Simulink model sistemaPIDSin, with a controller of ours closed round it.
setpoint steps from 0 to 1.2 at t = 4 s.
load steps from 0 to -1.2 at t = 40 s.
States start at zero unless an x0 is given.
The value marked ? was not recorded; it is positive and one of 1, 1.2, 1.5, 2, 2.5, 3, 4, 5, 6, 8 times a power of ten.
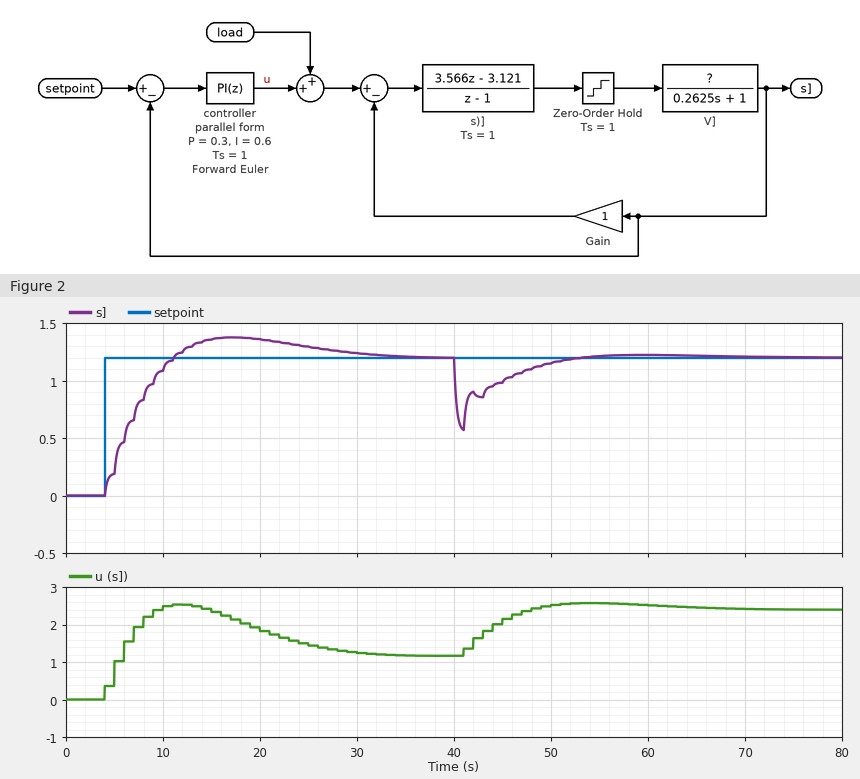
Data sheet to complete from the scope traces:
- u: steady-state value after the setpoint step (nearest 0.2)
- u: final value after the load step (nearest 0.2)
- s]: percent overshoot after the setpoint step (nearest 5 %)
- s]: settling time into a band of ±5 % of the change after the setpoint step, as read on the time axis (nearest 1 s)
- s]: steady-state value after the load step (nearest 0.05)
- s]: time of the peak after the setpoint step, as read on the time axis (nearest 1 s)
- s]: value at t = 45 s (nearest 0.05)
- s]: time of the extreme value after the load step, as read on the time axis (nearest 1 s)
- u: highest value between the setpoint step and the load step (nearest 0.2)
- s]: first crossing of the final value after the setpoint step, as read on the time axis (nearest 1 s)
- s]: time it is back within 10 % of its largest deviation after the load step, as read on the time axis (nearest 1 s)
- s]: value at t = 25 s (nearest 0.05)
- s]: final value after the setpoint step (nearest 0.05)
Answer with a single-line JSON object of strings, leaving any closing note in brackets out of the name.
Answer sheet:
{"u: steady-state value after the setpoint step": "1.2", "u: final value after the load step": "2.4", "s]: percent overshoot after the setpoint step": "15 %", "s]: settling time into a band of ±5 % of the change after the setpoint step, as read on the time axis": "28 s", "s]: steady-state value after the load step": "1.20", "s]: time of the peak after the setpoint step, as read on the time axis": "17 s", "s]: value at t = 45 s": "1.00", "s]: time of the extreme value after the load step, as read on the time axis": "41 s", "u: highest value between the setpoint step and the load step": "2.6", "s]: first crossing of the final value after the setpoint step, as read on the time axis": "11 s", "s]: time it is back within 10 % of its largest deviation after the load step, as read on the time axis": "49 s", "s]: value at t = 25 s": "1.30", "s]: final value after the setpoint step": "1.20"}
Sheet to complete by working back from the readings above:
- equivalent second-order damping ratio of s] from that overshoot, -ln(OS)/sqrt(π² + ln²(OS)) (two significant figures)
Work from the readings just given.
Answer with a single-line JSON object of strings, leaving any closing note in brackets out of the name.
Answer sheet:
{"equivalent second-order damping ratio of s] from that overshoot, -ln(OS)/sqrt(π² + ln²(OS))": "0.52"}
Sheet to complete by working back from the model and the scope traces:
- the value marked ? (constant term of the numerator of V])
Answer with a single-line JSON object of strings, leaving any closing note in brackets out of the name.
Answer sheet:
{"the value marked ?": "0.15"}
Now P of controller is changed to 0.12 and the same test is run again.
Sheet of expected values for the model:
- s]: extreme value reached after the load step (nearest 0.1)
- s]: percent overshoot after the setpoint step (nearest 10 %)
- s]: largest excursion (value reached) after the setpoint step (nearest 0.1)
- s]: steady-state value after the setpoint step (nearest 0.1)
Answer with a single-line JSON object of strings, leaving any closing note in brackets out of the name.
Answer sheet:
{"s]: extreme value reached after the load step": "0.6", "s]: percent overshoot after the setpoint step": "20 %", "s]: largest excursion (value reached) after the setpoint step": "1.4", "s]: steady-state value after the setpoint step": "1.2"}
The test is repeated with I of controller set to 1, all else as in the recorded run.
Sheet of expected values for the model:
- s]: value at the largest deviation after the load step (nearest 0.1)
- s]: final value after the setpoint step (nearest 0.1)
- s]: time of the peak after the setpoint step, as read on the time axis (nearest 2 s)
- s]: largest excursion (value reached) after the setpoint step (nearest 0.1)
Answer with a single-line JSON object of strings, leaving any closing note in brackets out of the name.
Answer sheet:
{"s]: value at the largest deviation after the load step": "0.6", "s]: final value after the setpoint step": "1.2", "s]: time of the peak after the setpoint step, as read on the time axis": "12 s", "s]: largest excursion (value reached) after the setpoint step": "1.4"}
